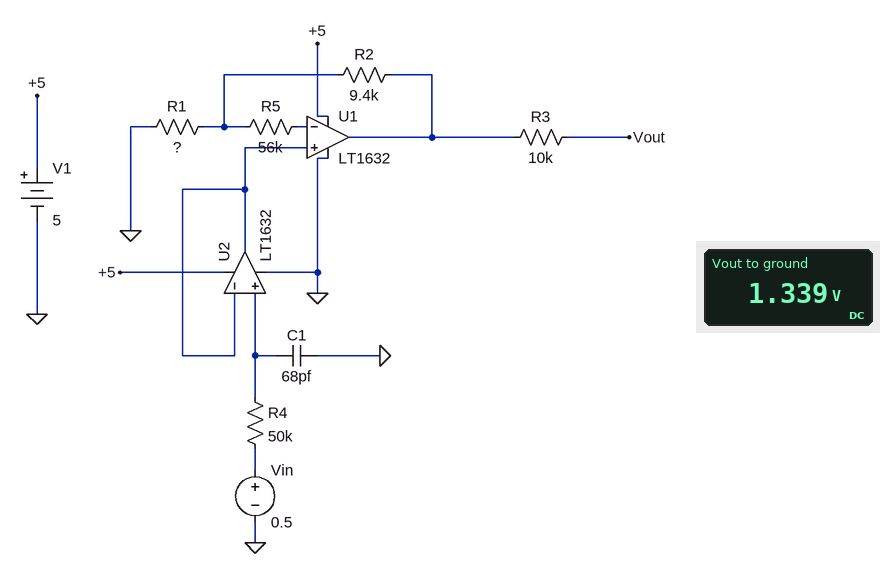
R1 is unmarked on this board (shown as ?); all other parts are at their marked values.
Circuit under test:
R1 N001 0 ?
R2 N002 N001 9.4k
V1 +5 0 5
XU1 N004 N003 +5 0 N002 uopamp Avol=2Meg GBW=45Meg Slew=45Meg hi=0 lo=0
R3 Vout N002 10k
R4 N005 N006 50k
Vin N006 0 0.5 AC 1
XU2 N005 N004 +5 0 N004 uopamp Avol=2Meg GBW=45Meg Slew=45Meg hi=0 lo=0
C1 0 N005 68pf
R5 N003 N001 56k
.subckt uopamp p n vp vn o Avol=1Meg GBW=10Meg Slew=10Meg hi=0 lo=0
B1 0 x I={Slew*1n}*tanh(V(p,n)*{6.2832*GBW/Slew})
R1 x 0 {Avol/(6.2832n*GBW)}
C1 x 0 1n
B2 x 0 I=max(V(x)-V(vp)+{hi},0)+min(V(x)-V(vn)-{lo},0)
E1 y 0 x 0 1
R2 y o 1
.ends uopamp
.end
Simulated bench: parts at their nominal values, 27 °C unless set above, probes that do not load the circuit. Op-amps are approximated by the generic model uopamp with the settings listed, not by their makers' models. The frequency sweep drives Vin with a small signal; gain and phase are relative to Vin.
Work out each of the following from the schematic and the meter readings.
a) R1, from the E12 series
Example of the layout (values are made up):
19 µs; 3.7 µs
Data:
5.6 kΩ
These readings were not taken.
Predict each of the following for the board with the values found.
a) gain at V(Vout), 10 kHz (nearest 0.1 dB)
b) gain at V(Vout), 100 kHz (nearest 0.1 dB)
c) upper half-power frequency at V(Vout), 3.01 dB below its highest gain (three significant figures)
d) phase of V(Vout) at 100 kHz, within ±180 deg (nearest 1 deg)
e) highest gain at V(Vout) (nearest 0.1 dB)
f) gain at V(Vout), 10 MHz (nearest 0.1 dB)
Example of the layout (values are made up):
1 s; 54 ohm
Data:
8.4 dB; 1.1 dB; 46.8 kHz; -65 deg; 8.6 dB; -39.6 dB
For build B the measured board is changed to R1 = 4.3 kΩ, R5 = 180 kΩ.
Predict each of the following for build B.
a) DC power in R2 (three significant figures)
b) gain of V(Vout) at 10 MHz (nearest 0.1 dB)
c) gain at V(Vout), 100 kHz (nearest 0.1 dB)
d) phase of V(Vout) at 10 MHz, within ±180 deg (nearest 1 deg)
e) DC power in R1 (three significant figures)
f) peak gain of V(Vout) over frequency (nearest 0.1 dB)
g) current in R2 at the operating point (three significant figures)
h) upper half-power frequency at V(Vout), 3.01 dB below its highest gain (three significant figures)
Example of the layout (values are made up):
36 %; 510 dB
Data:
127 µW; -38.5 dB; 2.6 dB; -138 deg; 58.1 µW; 10.1 dB; 116 µA; 46.8 kHz
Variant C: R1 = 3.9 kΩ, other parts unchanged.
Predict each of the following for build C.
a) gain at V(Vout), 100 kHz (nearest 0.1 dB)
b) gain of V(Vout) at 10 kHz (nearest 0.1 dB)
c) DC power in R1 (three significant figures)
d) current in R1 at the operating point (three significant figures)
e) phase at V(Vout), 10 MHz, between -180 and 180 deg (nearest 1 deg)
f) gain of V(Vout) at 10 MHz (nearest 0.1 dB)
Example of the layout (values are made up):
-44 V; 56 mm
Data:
3.2 dB; 10.5 dB; 64.1 µW; 128 µA; -139 deg; -38.1 dB
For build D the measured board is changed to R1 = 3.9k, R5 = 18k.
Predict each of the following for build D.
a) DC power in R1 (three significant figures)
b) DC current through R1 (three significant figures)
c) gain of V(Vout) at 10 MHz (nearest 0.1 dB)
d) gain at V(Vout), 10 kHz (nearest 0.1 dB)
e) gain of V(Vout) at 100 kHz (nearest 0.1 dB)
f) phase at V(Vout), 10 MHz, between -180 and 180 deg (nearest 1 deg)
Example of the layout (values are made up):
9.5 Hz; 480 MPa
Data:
64.1 µW; 128 µA; -38.1 dB; 10.5 dB; 3.2 dB; -139 deg
